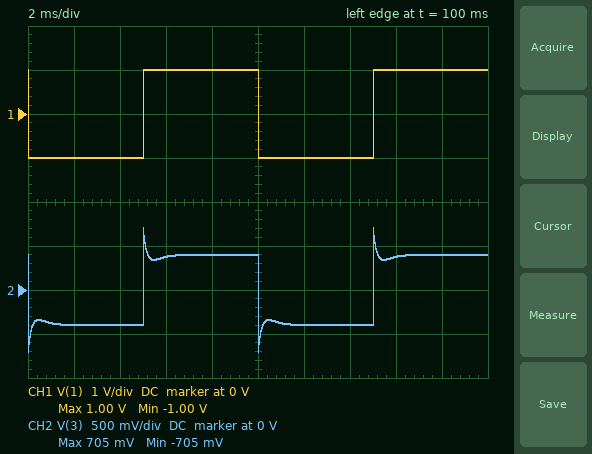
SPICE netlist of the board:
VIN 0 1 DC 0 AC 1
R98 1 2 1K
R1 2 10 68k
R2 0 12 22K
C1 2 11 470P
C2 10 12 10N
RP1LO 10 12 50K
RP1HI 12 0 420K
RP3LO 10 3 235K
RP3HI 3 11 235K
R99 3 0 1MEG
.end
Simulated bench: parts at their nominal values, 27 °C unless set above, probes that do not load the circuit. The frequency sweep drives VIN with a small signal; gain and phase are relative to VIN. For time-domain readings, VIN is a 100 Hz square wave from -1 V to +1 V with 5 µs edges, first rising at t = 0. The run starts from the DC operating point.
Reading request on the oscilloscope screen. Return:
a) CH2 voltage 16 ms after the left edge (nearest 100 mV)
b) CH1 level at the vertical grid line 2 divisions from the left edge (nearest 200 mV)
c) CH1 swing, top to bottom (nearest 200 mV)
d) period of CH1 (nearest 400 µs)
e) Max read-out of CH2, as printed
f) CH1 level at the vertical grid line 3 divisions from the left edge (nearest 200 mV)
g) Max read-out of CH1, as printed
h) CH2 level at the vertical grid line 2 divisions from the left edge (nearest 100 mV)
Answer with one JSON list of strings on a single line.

["400 mV", "-1.0 V", "2.0 V", "10.0 ms", "705 mV", "1.0 V", "1.00 V", "-400 mV"]
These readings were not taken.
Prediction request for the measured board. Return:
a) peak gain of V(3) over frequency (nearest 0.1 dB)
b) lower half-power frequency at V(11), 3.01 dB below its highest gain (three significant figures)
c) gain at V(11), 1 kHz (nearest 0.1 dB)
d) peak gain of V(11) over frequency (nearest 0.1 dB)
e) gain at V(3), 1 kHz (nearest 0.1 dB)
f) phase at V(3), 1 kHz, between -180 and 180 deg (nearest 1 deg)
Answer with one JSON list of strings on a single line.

["-5.1 dB", "878 Hz", "-2.6 dB", "-0.1 dB", "-7.0 dB", "-166 deg"]
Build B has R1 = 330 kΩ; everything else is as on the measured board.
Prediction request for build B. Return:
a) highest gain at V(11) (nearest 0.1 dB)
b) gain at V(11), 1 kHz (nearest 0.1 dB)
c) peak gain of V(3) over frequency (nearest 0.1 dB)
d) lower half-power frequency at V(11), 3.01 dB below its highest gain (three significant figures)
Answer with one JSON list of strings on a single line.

["0 dB", "-2.3 dB", "-6.3 dB", "828 Hz"]
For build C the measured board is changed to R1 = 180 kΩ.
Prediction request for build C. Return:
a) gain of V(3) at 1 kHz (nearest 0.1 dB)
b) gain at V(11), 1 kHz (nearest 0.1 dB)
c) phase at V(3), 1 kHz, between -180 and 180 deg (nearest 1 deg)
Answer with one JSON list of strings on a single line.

["-8.2 dB", "-2.4 dB", "-156 deg"]
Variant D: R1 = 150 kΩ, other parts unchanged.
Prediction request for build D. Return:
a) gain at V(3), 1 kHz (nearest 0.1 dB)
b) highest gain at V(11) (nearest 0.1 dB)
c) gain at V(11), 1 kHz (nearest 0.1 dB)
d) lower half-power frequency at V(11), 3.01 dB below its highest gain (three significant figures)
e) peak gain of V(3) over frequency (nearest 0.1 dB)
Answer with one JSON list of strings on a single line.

["-8.0 dB", "-0.1 dB", "-2.5 dB", "860 Hz", "-5.8 dB"]
